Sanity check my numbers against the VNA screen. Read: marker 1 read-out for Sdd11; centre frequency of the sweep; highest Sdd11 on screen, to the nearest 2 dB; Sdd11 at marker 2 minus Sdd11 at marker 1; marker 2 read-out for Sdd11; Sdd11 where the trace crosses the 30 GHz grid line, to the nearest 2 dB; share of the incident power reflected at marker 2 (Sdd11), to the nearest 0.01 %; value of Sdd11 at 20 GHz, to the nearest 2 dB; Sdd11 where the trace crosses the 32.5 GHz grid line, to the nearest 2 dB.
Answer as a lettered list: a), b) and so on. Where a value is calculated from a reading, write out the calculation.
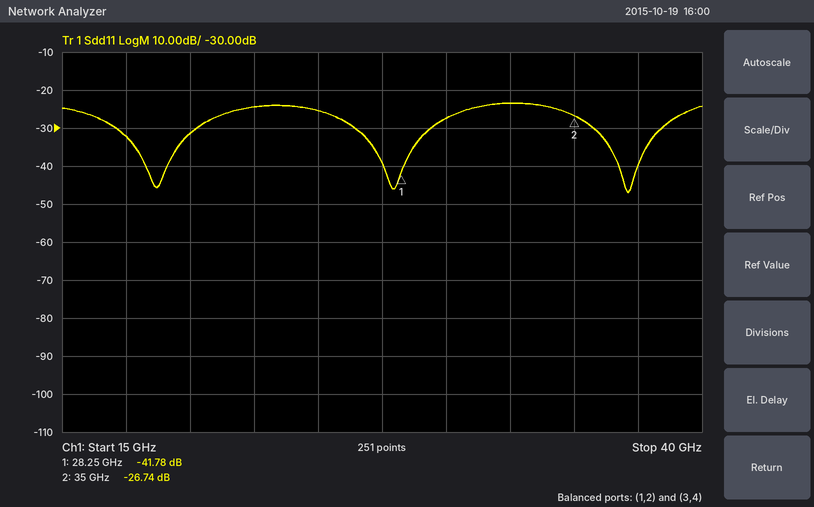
a) -41.78 dB
b) 27.5 GHz
c) -24 dB
d) -26.74 − (-41.78) = 15.04 dB
e) -26.74 dB
f) -28 dB
g) 10^(-26.74/10) ≈ 0.21 %
h) -32 dB
i) -24 dB
